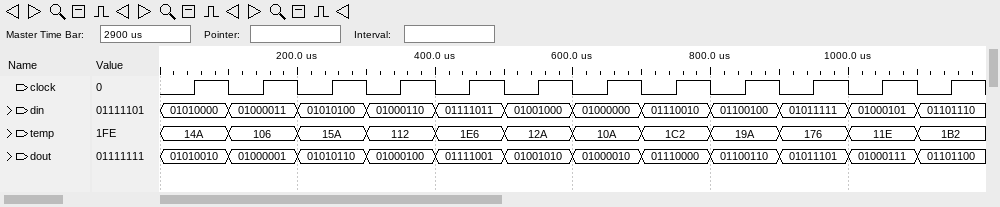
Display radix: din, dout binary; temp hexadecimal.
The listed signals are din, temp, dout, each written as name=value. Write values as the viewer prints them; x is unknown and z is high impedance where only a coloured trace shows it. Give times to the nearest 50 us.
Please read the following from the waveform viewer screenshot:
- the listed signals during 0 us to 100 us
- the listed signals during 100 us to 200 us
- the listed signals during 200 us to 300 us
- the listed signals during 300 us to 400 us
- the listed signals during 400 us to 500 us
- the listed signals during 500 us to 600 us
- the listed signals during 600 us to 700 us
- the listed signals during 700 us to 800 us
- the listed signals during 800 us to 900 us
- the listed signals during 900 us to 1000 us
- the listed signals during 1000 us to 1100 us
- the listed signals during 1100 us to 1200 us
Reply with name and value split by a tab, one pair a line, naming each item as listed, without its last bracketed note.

the listed signals during 0 us to 100 us	din=01010000, temp=14A, dout=01010010
the listed signals during 100 us to 200 us	din=01000011, temp=106, dout=01000001
the listed signals during 200 us to 300 us	din=01010100, temp=15A, dout=01010110
the listed signals during 300 us to 400 us	din=01000110, temp=112, dout=01000100
the listed signals during 400 us to 500 us	din=01111011, temp=1E6, dout=01111001
the listed signals during 500 us to 600 us	din=01001000, temp=12A, dout=01001010
the listed signals during 600 us to 700 us	din=01000000, temp=10A, dout=01000010
the listed signals during 700 us to 800 us	din=01110010, temp=1C2, dout=01110000
the listed signals during 800 us to 900 us	din=01100100, temp=19A, dout=01100110
the listed signals during 900 us to 1000 us	din=01011111, temp=176, dout=01011101
the listed signals during 1000 us to 1100 us	din=01000101, temp=11E, dout=01000111
the listed signals during 1100 us to 1200 us	din=01101110, temp=1B2, dout=01101100
